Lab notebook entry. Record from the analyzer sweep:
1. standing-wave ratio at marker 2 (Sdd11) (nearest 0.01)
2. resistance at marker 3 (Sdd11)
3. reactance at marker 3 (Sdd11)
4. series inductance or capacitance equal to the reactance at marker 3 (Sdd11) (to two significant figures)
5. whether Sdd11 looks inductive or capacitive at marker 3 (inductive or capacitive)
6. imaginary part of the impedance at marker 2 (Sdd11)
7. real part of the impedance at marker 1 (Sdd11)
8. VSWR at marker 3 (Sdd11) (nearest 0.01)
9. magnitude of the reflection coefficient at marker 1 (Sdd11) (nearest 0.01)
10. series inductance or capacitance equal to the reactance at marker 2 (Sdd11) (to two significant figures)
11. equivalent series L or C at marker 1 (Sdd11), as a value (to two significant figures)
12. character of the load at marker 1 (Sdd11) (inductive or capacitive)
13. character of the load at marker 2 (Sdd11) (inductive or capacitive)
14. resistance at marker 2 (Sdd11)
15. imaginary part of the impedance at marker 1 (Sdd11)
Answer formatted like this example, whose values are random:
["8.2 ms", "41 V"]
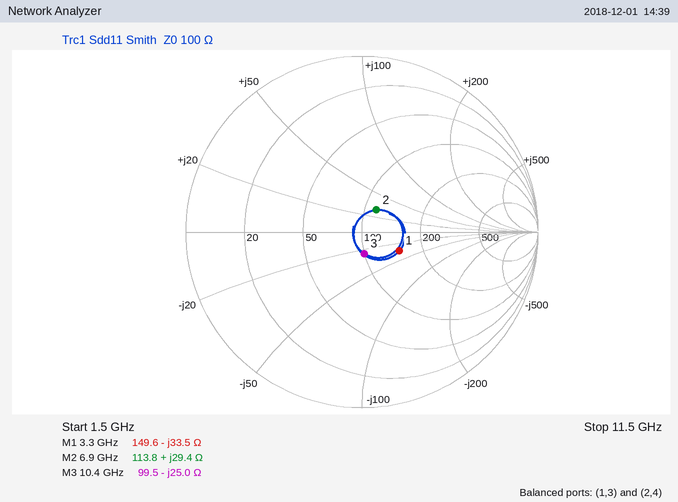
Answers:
["1.35", "99.5 Ω", "-25.0 Ω", "610 fF", "capacitive", "+29.4 Ω", "149.6 Ω", "1.28", "0.24", "680 pH", "1.4 pF", "capacitive", "inductive", "113.8 Ω", "-33.5 Ω"]
